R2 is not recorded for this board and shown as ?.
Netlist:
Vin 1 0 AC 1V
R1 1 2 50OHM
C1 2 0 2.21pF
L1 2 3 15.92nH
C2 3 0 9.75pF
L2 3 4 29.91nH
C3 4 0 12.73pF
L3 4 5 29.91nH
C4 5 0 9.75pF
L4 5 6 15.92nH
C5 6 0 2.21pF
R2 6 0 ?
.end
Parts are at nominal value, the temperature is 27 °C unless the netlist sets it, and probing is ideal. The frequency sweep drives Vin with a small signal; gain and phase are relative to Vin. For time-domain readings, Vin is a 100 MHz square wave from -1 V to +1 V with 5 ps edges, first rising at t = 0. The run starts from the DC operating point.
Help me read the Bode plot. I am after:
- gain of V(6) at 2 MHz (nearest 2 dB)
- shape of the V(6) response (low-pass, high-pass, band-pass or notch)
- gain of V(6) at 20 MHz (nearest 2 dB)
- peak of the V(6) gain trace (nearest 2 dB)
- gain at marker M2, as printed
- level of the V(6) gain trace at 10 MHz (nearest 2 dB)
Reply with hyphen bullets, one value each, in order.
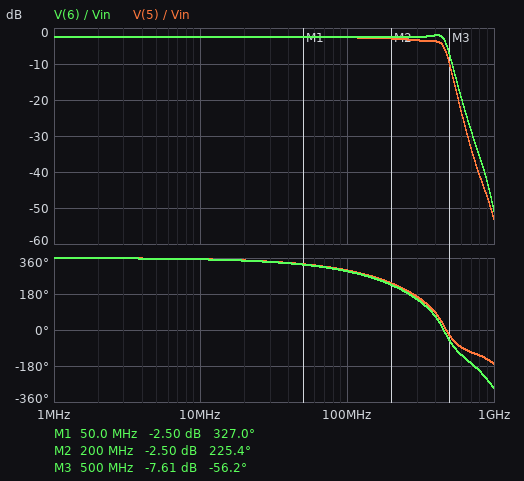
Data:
- -2 dB
- low-pass
- -2 dB
- -2 dB
- -2.50 dB
- -2 dB
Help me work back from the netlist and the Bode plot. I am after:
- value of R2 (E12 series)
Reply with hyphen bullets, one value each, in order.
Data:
- 150 Ω
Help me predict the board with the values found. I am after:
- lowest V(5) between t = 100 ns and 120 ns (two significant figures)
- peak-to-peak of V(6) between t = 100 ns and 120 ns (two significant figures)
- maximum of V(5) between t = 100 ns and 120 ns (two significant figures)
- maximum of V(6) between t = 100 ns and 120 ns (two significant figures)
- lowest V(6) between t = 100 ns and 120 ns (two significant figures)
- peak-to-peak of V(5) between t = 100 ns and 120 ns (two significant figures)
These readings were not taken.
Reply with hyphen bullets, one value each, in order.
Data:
- -940 mV
- 2.0 V
- 940 mV
- 1.0 V
- -1.0 V
- 1.9 V
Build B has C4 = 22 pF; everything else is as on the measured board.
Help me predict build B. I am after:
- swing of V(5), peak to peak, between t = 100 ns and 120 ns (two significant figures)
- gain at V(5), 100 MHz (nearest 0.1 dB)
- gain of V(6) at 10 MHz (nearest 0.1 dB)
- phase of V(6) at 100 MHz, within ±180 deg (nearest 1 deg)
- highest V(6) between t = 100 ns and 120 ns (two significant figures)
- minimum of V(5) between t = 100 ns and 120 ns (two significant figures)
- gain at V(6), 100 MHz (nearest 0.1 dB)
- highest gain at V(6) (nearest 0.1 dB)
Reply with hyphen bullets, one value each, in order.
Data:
- 1.5 V
- -3.2 dB
- -2.5 dB
- -82 deg
- 780 mV
- -770 mV
- -3.1 dB
- -2.5 dB
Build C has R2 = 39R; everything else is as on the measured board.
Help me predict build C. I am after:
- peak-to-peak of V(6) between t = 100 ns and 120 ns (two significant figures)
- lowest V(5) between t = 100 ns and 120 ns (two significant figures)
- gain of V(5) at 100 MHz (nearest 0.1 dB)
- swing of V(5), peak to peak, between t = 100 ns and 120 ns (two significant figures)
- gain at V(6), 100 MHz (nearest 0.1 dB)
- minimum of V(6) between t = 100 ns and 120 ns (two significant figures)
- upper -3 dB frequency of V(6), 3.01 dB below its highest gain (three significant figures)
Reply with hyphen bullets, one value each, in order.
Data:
- 1.2 V
- -680 mV
- -7.0 dB
- 1.4 V
- -7.2 dB
- -600 mV
- 508 MHz
